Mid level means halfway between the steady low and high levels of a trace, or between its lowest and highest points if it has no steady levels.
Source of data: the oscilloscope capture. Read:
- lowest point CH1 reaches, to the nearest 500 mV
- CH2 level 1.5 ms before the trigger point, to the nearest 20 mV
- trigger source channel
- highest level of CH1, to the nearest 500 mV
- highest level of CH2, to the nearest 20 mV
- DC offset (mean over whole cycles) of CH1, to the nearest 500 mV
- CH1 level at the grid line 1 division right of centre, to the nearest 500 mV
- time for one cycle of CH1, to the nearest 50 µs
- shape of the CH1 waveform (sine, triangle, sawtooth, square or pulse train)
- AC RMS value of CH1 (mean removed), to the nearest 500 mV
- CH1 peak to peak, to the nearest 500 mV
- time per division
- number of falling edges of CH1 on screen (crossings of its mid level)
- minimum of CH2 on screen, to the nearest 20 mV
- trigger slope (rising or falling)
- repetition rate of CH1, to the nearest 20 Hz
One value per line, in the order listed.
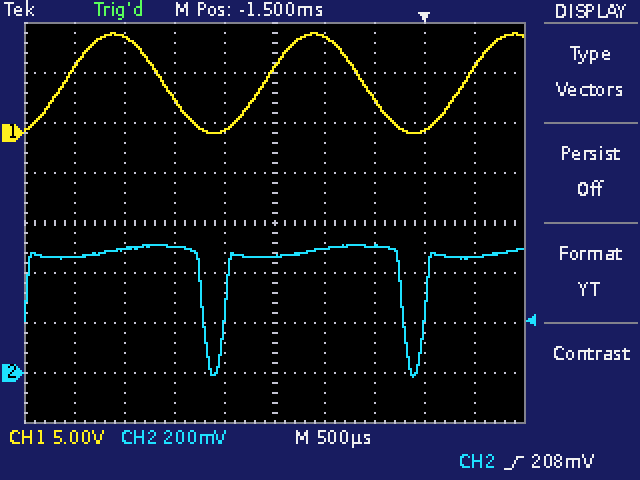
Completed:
0.0 V
460 mV
CH2
10.0 V
520 mV
5.0 V
9.5 V
2.00 ms
sine
3.5 V
10.0 V
500 µs
2
-20 mV
rising
500 Hz
